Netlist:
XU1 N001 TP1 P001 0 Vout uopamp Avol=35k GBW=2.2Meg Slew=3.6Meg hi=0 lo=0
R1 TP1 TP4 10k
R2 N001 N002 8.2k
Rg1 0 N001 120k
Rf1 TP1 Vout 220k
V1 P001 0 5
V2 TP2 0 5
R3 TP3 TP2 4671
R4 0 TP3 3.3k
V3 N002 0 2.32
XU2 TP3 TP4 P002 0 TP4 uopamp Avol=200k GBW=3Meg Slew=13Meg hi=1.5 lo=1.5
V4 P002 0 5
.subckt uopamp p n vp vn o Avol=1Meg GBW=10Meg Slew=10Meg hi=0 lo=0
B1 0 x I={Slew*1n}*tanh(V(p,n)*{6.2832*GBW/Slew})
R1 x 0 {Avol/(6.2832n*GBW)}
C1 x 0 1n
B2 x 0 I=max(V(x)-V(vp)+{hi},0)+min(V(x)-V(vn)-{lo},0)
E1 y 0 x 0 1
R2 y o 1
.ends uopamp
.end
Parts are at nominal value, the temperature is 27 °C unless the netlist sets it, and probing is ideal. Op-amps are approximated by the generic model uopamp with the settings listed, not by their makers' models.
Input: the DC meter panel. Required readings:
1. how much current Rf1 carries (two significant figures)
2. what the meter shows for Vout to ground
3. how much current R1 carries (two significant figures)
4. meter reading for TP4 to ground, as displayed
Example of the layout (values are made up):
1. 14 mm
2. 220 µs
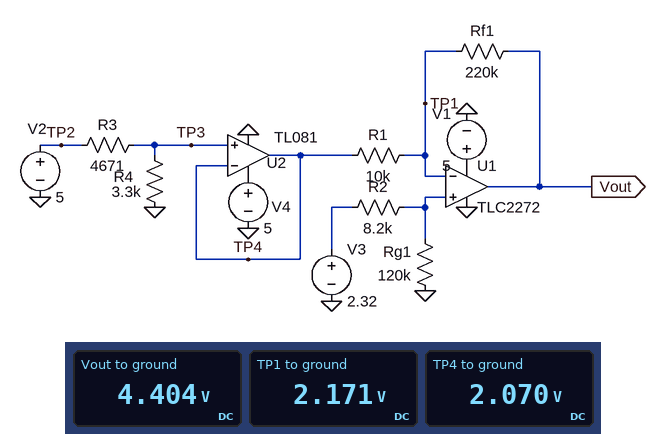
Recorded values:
1. 10 µA
2. 4.404 V
3. 10 µA
4. 2.070 V
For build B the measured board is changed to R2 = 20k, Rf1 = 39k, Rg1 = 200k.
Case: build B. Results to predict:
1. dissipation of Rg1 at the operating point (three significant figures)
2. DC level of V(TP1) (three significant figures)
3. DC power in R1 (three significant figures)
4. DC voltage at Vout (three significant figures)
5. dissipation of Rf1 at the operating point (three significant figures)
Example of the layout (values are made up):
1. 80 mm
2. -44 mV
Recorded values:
1. 22.2 µW
2. 2.11 V
3. 152 nW
4. 2.26 V
5. 594 nW
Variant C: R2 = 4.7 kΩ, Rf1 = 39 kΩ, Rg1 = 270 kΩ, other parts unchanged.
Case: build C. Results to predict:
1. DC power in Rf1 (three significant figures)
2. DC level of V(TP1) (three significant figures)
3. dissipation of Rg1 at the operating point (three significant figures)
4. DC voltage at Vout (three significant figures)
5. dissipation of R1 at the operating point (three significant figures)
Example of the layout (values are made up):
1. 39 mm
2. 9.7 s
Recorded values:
1. 17.2 µW
2. 2.28 V
3. 19.3 µW
4. 3.10 V
5. 4.42 µW
